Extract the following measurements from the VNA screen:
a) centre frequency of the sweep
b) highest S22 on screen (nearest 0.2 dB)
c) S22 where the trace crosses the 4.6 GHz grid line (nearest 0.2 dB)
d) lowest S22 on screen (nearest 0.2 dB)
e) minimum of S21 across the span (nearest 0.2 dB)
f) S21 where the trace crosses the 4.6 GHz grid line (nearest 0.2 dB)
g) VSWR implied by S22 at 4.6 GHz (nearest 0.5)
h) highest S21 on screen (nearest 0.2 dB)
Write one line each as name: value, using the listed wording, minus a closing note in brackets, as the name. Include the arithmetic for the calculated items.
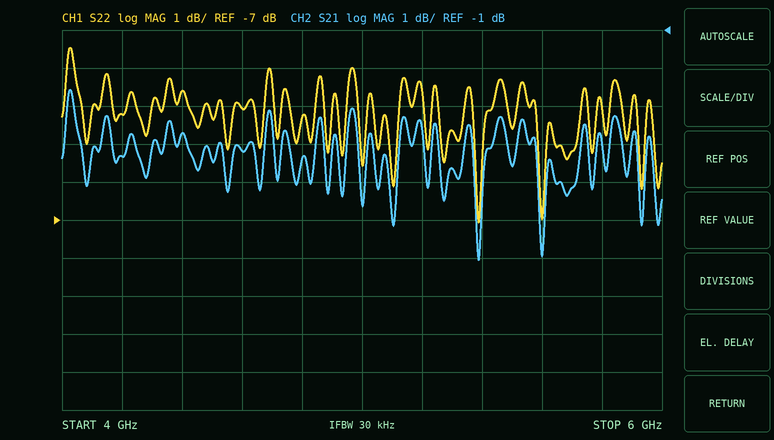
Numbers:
centre frequency of the sweep: 5 GHz
highest S22 on screen: -2.4 dB
S22 where the trace crosses the 4.6 GHz grid line: -4.0 dB
lowest S22 on screen: -7.0 dB
minimum of S21 across the span: -7.0 dB
S21 where the trace crosses the 4.6 GHz grid line: -4.2 dB
VSWR implied by S22 at 4.6 GHz: |Γ| = 10^(-4/20) = 0.6310; VSWR = (1 + 0.6310)/(1 − 0.6310) ≈ 4.42, so 4.5 to the nearest 0.5
highest S21 on screen: -2.6 dB
